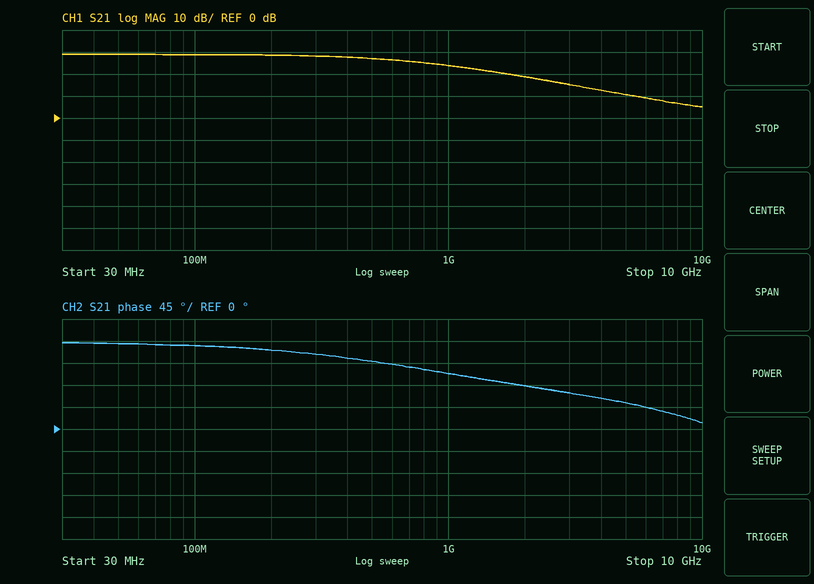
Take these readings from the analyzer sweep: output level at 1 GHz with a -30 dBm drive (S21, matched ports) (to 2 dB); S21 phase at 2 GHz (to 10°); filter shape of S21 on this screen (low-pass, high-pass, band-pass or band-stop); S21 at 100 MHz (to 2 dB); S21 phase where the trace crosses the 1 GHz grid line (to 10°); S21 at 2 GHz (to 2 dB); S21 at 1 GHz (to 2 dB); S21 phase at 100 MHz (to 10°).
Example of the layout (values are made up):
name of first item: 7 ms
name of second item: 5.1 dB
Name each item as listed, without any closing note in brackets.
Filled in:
output level at 1 GHz with a -30 dBm drive (S21, matched ports): -6 dBm
S21 phase at 2 GHz: 90°
filter shape of S21 on this screen: low-pass
S21 at 100 MHz: 28 dB
S21 phase where the trace crosses the 1 GHz grid line: 110°
S21 at 2 GHz: 18 dB
S21 at 1 GHz: 24 dB
S21 phase at 100 MHz: 170°
